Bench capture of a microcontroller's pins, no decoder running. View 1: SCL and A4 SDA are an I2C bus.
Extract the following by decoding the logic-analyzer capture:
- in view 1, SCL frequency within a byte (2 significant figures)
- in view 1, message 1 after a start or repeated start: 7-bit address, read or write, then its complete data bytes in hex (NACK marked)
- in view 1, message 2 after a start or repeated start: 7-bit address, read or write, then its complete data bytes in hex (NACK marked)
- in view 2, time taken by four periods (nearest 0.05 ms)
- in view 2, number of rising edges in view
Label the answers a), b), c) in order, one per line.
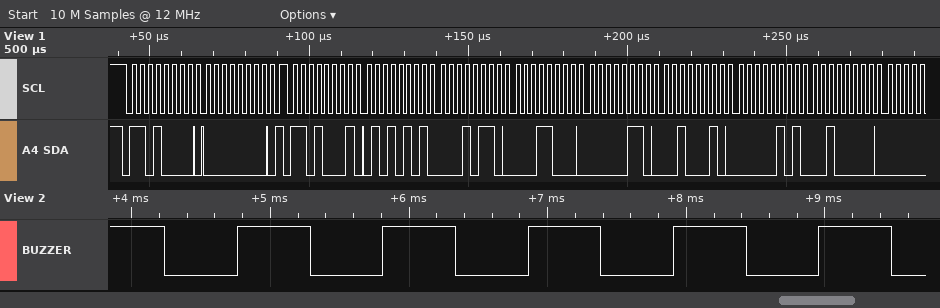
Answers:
a) 400 kHz
b) 0x68 write: 00
c) 0x68 read: 55 16 18 06 22 05 20
d) 4.20 ms
e) 5
